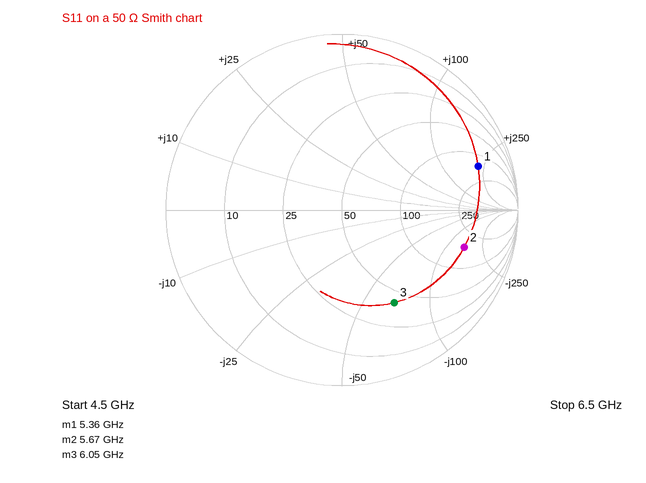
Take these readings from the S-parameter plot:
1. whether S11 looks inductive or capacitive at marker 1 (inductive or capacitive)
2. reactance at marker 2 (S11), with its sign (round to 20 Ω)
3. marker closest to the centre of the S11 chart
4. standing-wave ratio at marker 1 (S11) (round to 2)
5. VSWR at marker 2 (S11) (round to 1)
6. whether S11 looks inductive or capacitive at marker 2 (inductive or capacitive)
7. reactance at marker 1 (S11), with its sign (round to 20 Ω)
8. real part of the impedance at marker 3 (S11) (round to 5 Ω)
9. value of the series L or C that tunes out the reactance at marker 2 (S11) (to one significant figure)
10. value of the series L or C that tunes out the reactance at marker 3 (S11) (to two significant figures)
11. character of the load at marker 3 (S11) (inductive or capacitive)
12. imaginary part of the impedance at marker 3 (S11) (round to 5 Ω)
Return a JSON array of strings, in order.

["inductive", "-160 Ω", "marker 3", "10", "6", "capacitive", "+220 Ω", "40 Ω", "4 nH", "1.8 nH", "capacitive", "-70 Ω"]
